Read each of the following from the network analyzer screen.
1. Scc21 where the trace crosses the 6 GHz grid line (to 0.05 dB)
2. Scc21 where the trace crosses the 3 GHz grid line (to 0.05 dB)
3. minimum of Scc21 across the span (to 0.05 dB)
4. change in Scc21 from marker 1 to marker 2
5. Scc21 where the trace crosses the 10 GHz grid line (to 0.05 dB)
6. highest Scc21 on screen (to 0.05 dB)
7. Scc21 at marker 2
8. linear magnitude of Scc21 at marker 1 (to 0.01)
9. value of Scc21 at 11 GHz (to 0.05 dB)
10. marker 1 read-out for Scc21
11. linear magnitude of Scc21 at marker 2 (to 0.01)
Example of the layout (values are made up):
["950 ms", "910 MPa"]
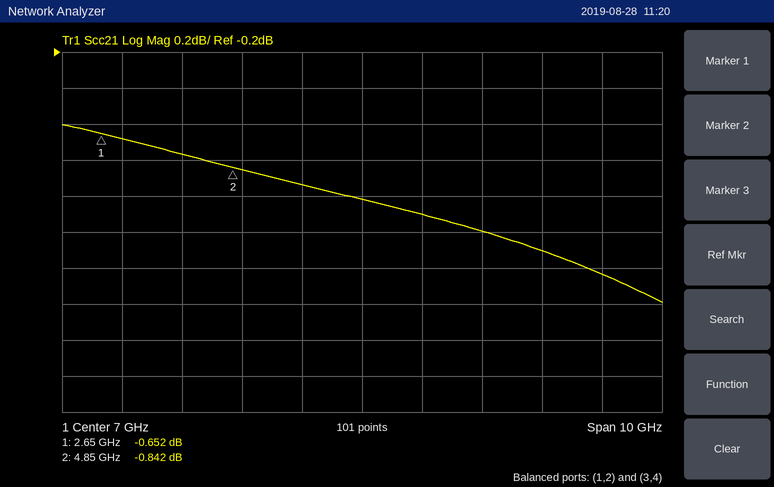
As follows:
["-0.95 dB", "-0.70 dB", "-1.60 dB", "-0.190 dB", "-1.30 dB", "-0.60 dB", "-0.842 dB", "0.93", "-1.45 dB", "-0.652 dB", "0.91"]
